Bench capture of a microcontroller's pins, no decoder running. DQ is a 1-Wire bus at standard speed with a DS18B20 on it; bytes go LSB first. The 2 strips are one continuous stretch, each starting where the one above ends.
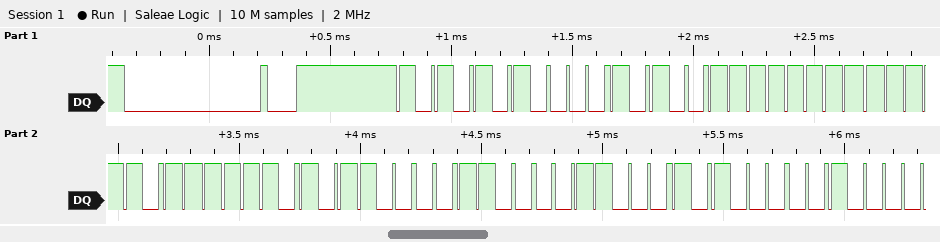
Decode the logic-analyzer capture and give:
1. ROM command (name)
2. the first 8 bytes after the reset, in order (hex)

Match ROM
55 28 FF DF AF 61 18 05
